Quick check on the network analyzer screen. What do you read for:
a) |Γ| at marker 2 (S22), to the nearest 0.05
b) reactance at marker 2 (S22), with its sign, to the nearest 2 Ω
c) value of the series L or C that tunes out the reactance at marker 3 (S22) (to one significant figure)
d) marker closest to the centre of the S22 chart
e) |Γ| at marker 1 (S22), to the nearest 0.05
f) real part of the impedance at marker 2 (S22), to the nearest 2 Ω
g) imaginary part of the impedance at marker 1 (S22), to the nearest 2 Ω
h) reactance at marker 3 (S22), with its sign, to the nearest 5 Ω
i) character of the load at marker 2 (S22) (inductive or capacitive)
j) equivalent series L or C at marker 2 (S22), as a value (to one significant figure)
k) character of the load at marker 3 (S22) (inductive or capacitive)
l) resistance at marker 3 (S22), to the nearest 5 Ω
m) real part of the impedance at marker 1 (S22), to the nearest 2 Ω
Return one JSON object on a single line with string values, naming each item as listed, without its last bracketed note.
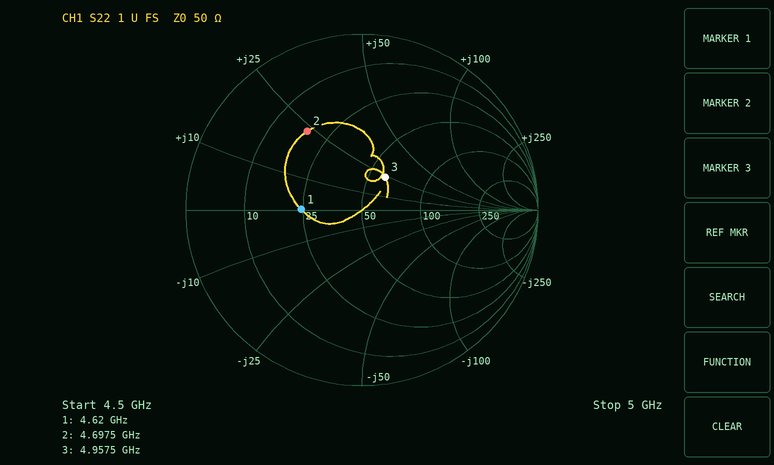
{"|Γ| at marker 2 (S22), to the nearest 0.05": "0.55", "reactance at marker 2 (S22), with its sign, to the nearest 2 Ω": "+24 Ω", "value of the series L or C that tunes out the reactance at marker 3 (S22)": "1 pF", "marker closest to the centre of the S22 chart": "marker 3", "|Γ| at marker 1 (S22), to the nearest 0.05": "0.35", "real part of the impedance at marker 2 (S22), to the nearest 2 Ω": "18 Ω", "imaginary part of the impedance at marker 1 (S22), to the nearest 2 Ω": "0 Ω", "reactance at marker 3 (S22), with its sign, to the nearest 5 Ω": "+25 Ω", "character of the load at marker 2 (S22)": "inductive", "equivalent series L or C at marker 2 (S22), as a value": "800 pH", "character of the load at marker 3 (S22)": "inductive", "resistance at marker 3 (S22), to the nearest 5 Ω": "60 Ω", "real part of the impedance at marker 1 (S22), to the nearest 2 Ω": "24 Ω"}
